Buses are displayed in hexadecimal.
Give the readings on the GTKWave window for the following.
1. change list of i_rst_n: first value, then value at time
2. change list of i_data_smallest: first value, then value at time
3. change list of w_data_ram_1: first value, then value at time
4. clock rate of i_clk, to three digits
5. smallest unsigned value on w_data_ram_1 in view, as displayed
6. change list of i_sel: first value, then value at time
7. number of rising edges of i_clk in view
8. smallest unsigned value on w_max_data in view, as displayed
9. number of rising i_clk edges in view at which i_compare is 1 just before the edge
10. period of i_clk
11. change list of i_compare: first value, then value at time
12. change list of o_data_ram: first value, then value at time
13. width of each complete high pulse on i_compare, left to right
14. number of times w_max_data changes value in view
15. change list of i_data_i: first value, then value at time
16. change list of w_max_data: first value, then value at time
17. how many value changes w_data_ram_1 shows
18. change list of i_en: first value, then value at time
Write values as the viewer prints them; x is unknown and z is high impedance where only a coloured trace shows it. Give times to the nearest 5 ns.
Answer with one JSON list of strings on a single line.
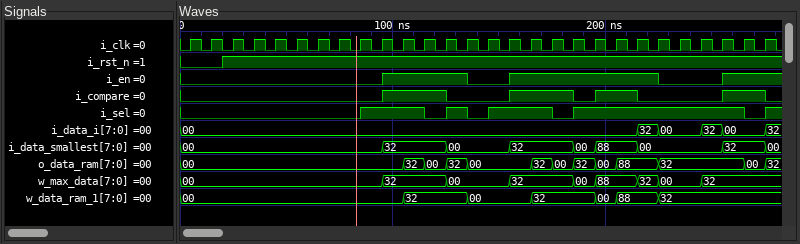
["0, 1 at 20 ns", "00, 32 at 95 ns, 00 at 125 ns, 32 at 155 ns, 00 at 185 ns, 88 at 195 ns, 00 at 215 ns, 32 at 255 ns, 00 at 275 ns", "00, 32 at 105 ns, 00 at 135 ns, 32 at 165 ns, 00 at 195 ns, 88 at 205 ns, 32 at 225 ns", "100 MHz", "00", "0, 1 at 85 ns, 0 at 115 ns, 1 at 125 ns, 0 at 135 ns, 1 at 145 ns, 0 at 175 ns, 1 at 185 ns, 0 at 265 ns, 1 at 275 ns", "28", "00", "10", "10 ns", "0, 1 at 95 ns, 0 at 125 ns, 1 at 155 ns, 0 at 185 ns, 1 at 195 ns, 0 at 215 ns, 1 at 255 ns, 0 at 275 ns", "00, 32 at 105 ns, 00 at 115 ns, 32 at 125 ns, 00 at 135 ns, 32 at 165 ns, 00 at 175 ns, 32 at 185 ns, 00 at 195 ns, 88 at 205 ns, 32 at 225 ns, 00 at 265 ns, 32 at 275 ns", "30 ns, 30 ns, 20 ns, 20 ns", "8", "00, 32 at 215 ns, 00 at 225 ns, 32 at 245 ns, 00 at 255 ns, 32 at 275 ns", "00, 32 at 95 ns, 00 at 125 ns, 32 at 155 ns, 00 at 185 ns, 88 at 195 ns, 32 at 215 ns, 00 at 225 ns, 32 at 245 ns", "6", "0, 1 at 95 ns, 0 at 135 ns, 1 at 155 ns, 0 at 225 ns, 1 at 255 ns"]
